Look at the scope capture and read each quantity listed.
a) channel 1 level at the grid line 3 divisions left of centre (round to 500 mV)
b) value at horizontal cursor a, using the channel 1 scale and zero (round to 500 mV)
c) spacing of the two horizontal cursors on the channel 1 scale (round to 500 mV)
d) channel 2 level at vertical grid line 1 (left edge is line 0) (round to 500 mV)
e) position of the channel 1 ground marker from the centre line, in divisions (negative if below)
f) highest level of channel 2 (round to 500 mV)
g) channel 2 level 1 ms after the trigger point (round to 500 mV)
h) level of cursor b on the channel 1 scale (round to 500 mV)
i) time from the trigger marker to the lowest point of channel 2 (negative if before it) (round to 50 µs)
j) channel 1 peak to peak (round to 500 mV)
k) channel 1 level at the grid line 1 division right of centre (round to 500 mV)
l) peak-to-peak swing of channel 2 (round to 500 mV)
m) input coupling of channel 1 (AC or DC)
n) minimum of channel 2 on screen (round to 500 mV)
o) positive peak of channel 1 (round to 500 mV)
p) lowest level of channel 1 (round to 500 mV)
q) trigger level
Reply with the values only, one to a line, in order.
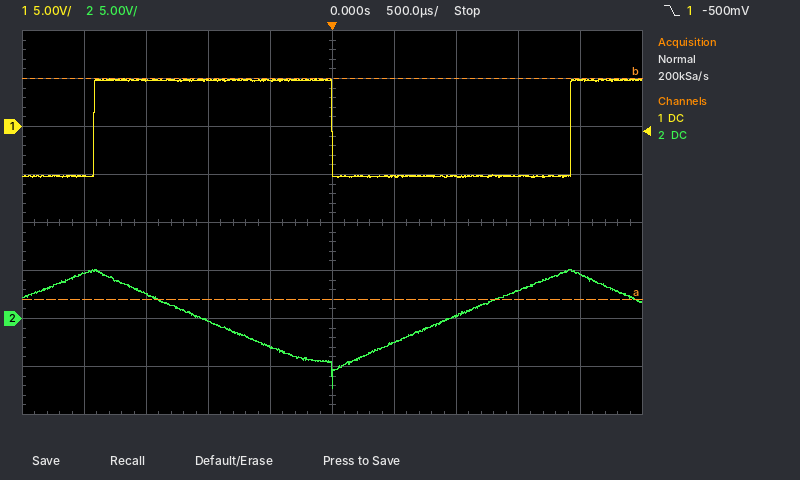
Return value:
5.0 V
-18.0 V
23.0 V
4.5 V
+2.0 div
5.0 V
500 mV
5.0 V
0 µs
10.5 V
-5.0 V
12.5 V
DC
-7.5 V
5.0 V
-5.5 V
-500 mV
